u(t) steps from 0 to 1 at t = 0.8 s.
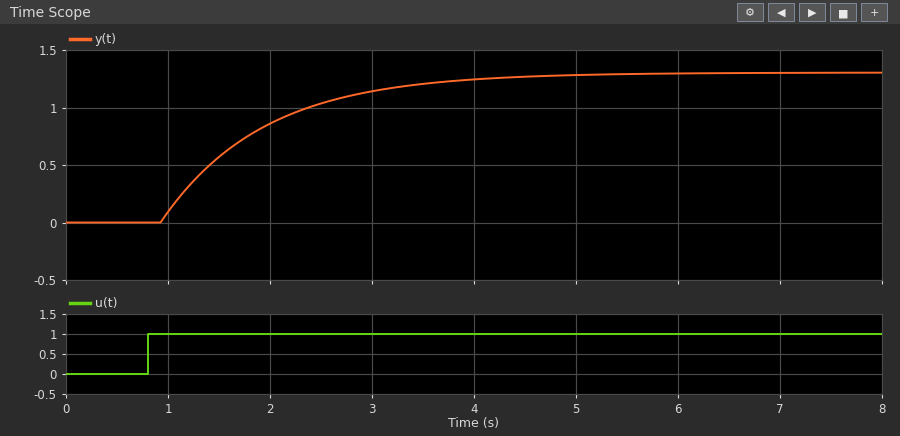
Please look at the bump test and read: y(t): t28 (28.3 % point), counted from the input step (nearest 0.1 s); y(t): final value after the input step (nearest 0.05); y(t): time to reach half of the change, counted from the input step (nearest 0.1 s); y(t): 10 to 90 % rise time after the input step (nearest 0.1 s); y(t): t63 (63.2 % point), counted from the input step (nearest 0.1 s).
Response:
0.5 s
1.30
0.8 s
2.2 s
1.1 s
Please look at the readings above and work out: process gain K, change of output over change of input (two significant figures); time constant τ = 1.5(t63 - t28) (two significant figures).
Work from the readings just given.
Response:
1.3
0.90 s
